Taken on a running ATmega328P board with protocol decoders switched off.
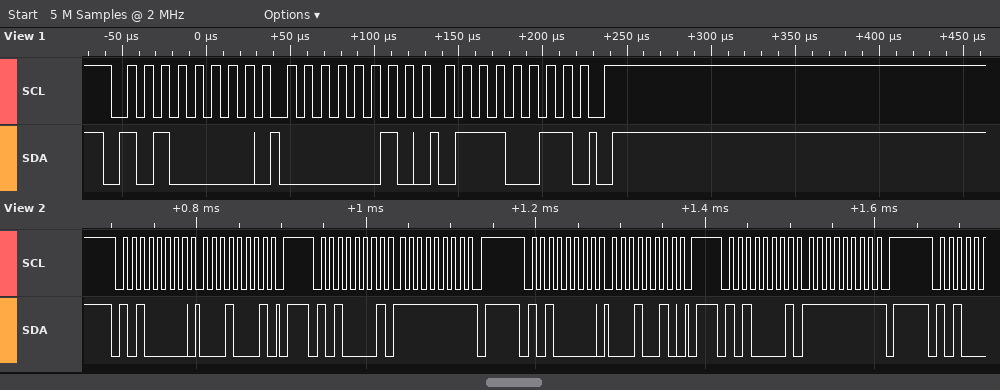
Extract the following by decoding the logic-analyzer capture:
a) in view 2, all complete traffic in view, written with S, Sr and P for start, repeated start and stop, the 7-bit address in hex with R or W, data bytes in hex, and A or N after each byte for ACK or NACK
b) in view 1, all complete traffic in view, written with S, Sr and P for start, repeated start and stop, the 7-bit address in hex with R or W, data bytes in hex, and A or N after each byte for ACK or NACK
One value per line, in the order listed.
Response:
S 50W A 11 A P S 50R A FF N P S 50W A 12 A P S 50R A FF N P
S 50W A 02 A 73 A P
